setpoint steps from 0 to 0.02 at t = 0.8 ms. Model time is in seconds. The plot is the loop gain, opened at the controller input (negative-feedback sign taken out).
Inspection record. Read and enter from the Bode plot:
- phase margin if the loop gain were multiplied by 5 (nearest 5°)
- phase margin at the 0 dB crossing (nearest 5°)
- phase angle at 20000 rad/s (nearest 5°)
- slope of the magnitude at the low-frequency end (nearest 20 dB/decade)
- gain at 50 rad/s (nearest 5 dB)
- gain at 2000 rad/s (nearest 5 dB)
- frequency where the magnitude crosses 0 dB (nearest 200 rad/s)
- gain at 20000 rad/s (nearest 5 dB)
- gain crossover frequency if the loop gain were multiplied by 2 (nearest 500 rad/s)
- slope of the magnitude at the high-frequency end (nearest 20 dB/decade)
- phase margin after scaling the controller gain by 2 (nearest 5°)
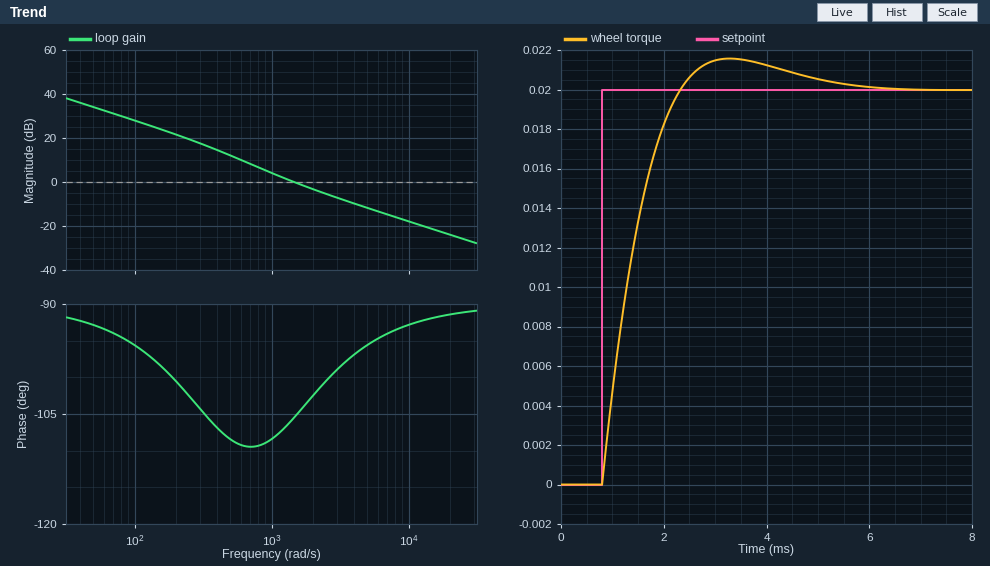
85°
75°
-90°
-20 dB/decade
35 dB
-5 dB
1400 rad/s
-25 dB
2500 rad/s
-20 dB/decade
80°
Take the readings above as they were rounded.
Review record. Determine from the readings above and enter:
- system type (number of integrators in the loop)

1
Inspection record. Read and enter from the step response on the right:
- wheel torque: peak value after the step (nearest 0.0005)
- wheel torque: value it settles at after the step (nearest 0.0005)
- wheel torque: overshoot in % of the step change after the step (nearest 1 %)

0.0215
0.0200
8 %
